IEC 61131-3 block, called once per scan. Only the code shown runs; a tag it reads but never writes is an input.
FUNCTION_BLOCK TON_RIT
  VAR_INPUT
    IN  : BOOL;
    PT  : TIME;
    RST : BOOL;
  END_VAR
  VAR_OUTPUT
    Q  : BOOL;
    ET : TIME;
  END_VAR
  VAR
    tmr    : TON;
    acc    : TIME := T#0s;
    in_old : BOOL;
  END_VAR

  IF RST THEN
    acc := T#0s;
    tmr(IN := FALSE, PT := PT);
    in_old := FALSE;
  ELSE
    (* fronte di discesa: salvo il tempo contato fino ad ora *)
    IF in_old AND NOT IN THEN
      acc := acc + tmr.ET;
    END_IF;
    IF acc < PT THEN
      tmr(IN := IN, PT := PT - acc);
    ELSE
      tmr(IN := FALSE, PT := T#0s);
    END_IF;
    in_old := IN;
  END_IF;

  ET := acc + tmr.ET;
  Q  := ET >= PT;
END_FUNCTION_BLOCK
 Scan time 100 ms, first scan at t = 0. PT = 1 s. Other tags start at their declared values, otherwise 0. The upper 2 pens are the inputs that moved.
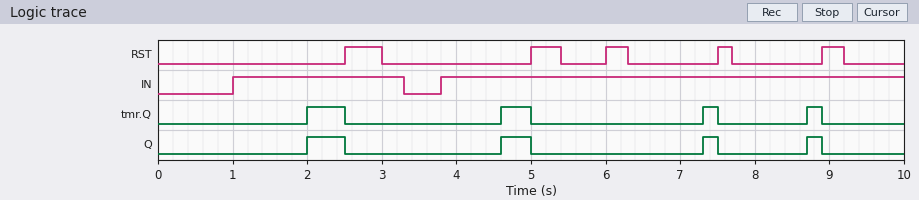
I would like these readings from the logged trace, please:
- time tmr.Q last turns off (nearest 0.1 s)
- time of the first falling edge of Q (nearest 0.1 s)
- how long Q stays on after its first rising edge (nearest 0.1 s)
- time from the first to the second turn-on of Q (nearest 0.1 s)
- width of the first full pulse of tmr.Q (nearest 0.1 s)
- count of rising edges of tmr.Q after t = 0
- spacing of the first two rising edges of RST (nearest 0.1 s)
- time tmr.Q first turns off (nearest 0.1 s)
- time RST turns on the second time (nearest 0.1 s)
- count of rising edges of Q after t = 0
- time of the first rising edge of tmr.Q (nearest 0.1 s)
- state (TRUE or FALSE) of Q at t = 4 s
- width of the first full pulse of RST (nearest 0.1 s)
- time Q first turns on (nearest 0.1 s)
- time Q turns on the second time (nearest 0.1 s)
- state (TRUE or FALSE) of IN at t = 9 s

8.9 s
2.5 s
0.5 s
2.6 s
0.5 s
4
2.5 s
2.5 s
5.0 s
4
2.0 s
FALSE
0.5 s
2.0 s
4.6 s
TRUE
